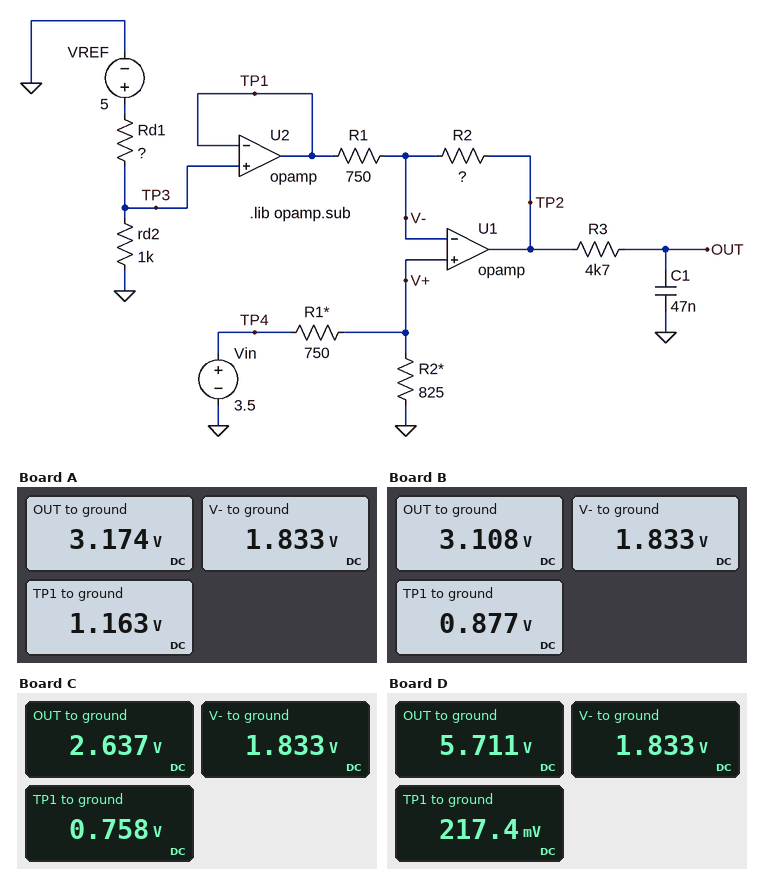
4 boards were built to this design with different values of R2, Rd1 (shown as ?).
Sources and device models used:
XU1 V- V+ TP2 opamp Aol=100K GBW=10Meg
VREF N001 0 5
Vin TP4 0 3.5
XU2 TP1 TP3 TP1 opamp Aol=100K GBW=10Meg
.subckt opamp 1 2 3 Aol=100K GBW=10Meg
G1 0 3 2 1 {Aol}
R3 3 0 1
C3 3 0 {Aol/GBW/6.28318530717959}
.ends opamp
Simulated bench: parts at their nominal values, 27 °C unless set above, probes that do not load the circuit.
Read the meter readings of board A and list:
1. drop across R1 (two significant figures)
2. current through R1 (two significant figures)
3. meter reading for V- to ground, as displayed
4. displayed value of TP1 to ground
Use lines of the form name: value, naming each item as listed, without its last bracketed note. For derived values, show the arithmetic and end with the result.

drop across R1: 1.833 V - 1.163 V = 670 mV
current through R1: (1.833 V - 1.163 V) / 750 Ω = 890 µA
meter reading for V- to ground, as displayed: 1.833 V
displayed value of TP1 to ground: 1.163 V
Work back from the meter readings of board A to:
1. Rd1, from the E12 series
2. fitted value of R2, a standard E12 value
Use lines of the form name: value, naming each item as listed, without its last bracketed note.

Rd1, from the E12 series: 3.3 kΩ
fitted value of R2, a standard E12 value: 1.5 kΩ
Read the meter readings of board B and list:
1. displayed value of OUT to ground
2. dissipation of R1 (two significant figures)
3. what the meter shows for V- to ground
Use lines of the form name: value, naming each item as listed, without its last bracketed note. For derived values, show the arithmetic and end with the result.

displayed value of OUT to ground: 3.108 V
dissipation of R1: (1.833 V - 877 mV)^2 / 750 Ω = 1.2 mW
what the meter shows for V- to ground: 1.833 V
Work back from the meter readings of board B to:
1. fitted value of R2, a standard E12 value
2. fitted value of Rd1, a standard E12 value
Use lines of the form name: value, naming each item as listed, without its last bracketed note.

fitted value of R2, a standard E12 value: 1 kΩ
fitted value of Rd1, a standard E12 value: 4.7 kΩ
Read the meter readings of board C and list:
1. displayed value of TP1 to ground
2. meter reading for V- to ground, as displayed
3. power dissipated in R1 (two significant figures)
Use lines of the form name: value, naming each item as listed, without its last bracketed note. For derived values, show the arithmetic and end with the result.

displayed value of TP1 to ground: 0.758 V
meter reading for V- to ground, as displayed: 1.833 V
power dissipated in R1: (1.833 V - 758 mV)^2 / 750 Ω = 1.5 mW
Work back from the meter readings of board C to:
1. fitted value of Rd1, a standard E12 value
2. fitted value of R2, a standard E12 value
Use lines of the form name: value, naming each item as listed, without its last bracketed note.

fitted value of Rd1, a standard E12 value: 5.6 kΩ
fitted value of R2, a standard E12 value: 560 Ω
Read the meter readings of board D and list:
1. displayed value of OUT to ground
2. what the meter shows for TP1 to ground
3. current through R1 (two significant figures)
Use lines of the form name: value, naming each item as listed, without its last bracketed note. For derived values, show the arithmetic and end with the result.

displayed value of OUT to ground: 5.711 V
what the meter shows for TP1 to ground: 217.4 mV
current through R1: (1.833 V - 217.4 mV) / 750 Ω = 2.2 mA
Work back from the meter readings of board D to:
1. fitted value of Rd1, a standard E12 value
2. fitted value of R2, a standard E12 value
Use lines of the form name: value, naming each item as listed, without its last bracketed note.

fitted value of Rd1, a standard E12 value: 22 kΩ
fitted value of R2, a standard E12 value: 1.8 kΩ
